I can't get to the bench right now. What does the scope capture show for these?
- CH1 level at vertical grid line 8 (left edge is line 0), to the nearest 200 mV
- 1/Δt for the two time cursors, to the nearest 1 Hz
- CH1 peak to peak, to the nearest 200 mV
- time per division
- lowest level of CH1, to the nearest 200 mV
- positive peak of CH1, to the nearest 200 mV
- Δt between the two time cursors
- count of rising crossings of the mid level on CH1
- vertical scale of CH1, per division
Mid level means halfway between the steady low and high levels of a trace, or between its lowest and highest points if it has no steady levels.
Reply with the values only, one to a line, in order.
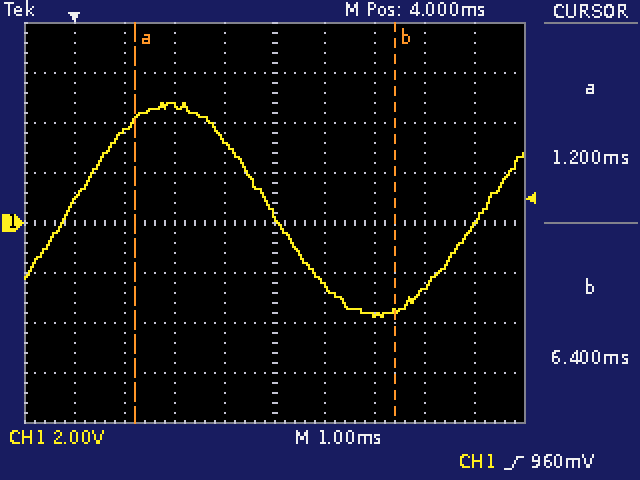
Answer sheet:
-2.6 V
192 Hz
8.6 V
1 ms
-3.8 V
4.8 V
5.2 ms
2
2 V
